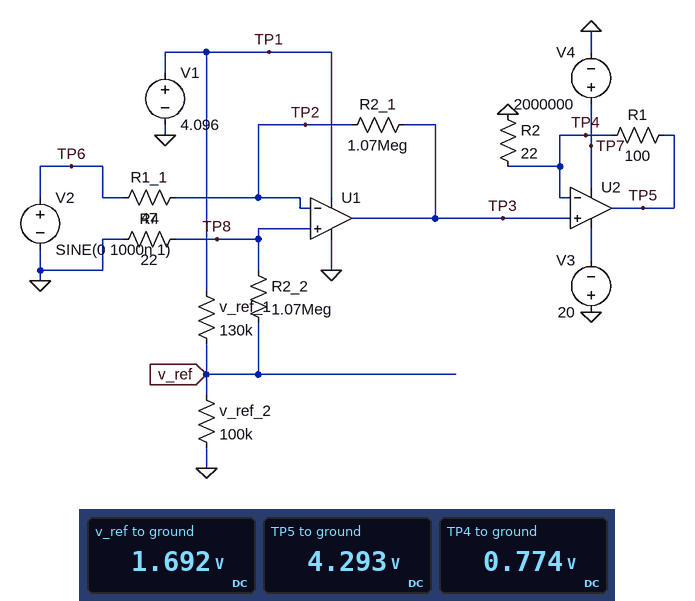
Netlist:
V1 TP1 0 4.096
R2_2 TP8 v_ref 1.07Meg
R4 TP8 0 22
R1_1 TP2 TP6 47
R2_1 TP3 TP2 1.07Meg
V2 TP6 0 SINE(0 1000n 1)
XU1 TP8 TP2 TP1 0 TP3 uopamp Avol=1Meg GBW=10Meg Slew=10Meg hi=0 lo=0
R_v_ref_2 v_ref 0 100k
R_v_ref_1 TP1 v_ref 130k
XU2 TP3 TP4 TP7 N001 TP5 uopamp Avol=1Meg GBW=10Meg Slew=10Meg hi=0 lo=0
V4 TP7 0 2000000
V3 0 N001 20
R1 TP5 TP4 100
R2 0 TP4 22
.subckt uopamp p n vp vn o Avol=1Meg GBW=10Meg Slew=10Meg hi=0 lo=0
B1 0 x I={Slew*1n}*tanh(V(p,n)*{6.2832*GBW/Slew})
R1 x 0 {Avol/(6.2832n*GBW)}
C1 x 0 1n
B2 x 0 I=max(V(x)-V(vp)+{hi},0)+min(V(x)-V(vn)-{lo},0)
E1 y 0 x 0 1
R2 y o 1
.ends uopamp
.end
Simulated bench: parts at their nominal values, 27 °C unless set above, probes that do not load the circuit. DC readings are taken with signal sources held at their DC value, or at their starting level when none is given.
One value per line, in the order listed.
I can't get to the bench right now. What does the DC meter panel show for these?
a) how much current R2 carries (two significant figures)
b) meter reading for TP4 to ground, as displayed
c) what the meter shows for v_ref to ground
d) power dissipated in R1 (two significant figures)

35 mA
0.774 V
1.692 V
120 mW
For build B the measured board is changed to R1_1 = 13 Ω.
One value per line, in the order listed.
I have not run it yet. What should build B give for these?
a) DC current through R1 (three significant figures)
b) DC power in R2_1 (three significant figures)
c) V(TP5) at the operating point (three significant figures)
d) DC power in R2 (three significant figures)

120 mA
6.54 µW
14.7 V
318 mW
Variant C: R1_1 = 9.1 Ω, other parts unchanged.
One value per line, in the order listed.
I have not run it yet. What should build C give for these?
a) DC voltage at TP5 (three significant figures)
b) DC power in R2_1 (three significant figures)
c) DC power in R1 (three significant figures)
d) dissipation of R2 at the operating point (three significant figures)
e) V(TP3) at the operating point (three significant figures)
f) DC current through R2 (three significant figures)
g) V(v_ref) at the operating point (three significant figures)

20.3 V
12.5 µW
2.77 W
609 mW
3.66 V
166 mA
1.69 V
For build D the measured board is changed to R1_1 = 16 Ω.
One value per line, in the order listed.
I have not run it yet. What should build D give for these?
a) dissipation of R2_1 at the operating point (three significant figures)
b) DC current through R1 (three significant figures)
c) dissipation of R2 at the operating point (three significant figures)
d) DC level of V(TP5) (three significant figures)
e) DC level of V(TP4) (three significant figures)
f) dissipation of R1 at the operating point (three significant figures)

4.44 µW
99.1 mA
216 mW
12.1 V
2.18 V
982 mW
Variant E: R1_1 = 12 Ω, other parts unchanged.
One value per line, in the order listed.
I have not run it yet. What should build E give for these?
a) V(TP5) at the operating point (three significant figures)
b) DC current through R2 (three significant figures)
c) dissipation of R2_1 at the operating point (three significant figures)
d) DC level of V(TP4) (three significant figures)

15.8 V
129 mA
7.58 µW
2.85 V
